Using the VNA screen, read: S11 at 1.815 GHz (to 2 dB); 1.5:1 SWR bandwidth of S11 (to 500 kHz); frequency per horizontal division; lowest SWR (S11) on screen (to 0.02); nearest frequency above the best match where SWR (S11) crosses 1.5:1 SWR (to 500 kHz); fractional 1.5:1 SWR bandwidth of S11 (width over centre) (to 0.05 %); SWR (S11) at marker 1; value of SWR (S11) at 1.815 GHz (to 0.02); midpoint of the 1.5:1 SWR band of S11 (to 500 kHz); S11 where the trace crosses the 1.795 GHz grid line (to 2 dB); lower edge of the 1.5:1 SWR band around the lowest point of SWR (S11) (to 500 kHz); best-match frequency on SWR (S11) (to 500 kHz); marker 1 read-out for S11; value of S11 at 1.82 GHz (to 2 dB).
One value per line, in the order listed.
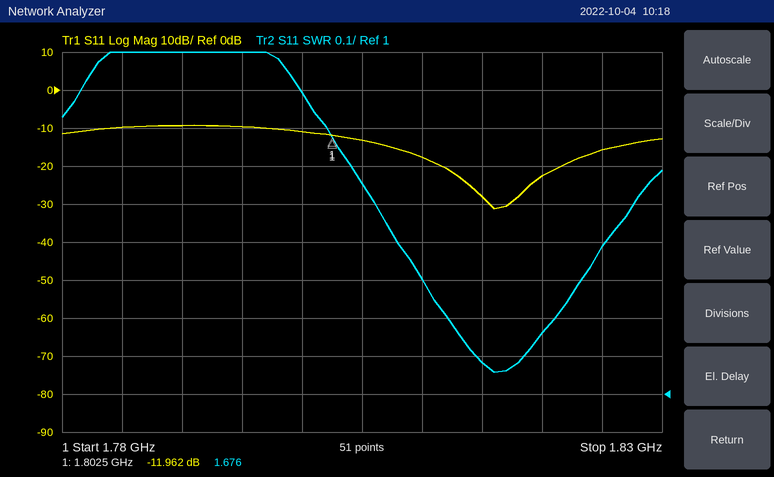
-28 dB
21.5 MHz
5 MHz
1.06
1.8275 GHz
1.20 %
1.676
1.08
1.8170 GHz
-10 dB
1.8060 GHz
1.8160 GHz
-11.962 dB
-22 dB
